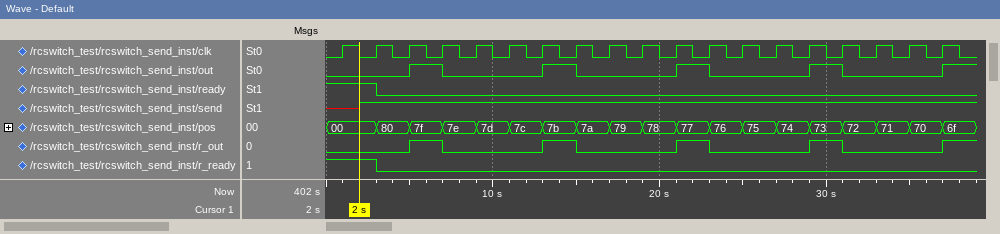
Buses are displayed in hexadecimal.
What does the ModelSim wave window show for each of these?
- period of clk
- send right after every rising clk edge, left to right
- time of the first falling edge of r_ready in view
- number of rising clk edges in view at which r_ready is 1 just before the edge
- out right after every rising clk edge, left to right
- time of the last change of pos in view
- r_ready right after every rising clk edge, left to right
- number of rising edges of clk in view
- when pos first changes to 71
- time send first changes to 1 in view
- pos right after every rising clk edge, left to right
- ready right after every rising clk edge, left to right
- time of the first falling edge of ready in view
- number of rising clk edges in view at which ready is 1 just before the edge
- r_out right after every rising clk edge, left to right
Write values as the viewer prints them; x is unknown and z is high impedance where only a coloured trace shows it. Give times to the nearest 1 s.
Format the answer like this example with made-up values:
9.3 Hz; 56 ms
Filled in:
2 s; x 1 1 1 1 1 1 1 1 1 1 1 1 1 1 1 1 1 1; 3 s; 2; 0 0 1 0 0 0 1 0 0 0 1 0 0 0 1 0 0 0 1; 37 s; 1 0 0 0 0 0 0 0 0 0 0 0 0 0 0 0 0 0 0; 19; 33 s; 2 s; 00, 80, 7f, 7e, 7d, 7c, 7b, 7a, 79, 78, 77, 76, 75, 74, 73, 72, 71, 70, 6f; 1 0 0 0 0 0 0 0 0 0 0 0 0 0 0 0 0 0 0; 3 s; 2; 0 0 1 0 0 0 1 0 0 0 1 0 0 0 1 0 0 0 1
